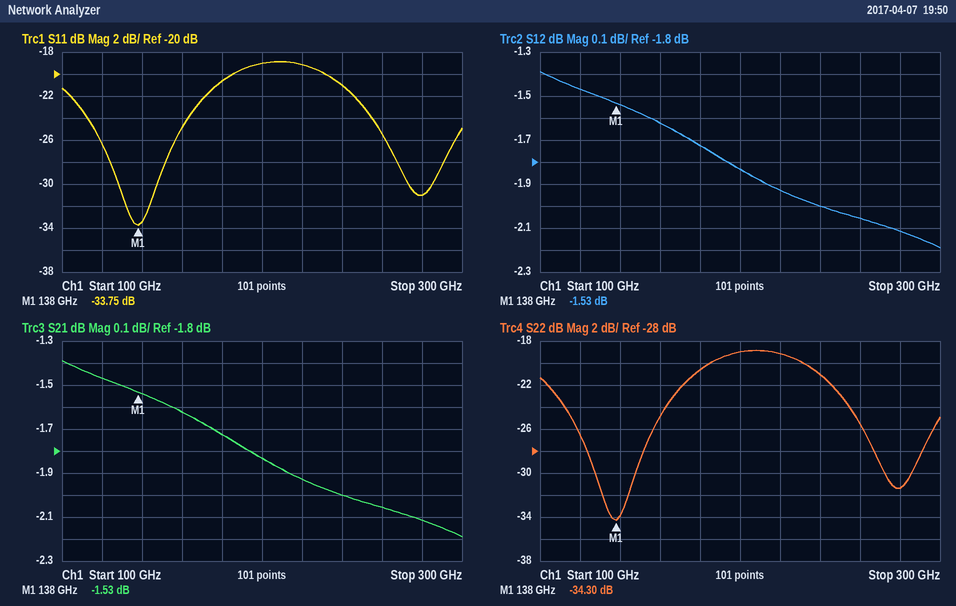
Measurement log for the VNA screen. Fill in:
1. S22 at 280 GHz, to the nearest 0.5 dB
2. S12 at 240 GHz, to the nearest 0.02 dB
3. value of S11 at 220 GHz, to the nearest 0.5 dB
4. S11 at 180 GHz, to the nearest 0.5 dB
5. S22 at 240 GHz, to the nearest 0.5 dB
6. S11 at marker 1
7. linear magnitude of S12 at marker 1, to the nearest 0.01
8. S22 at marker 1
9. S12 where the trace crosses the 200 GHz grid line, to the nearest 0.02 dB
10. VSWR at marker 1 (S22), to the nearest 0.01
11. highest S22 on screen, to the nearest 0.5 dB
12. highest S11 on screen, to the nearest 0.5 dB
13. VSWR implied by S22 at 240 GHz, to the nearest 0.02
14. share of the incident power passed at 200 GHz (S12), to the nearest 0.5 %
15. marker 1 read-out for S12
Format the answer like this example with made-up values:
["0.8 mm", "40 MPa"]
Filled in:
["-31.5 dB", "-2.00 dB", "-19.0 dB", "-20.5 dB", "-21.0 dB", "-33.75 dB", "0.84", "-34.30 dB", "-1.84 dB", "1.04", "-19.0 dB", "-19.0 dB", "1.20", "65.5 %", "-1.53 dB"]
